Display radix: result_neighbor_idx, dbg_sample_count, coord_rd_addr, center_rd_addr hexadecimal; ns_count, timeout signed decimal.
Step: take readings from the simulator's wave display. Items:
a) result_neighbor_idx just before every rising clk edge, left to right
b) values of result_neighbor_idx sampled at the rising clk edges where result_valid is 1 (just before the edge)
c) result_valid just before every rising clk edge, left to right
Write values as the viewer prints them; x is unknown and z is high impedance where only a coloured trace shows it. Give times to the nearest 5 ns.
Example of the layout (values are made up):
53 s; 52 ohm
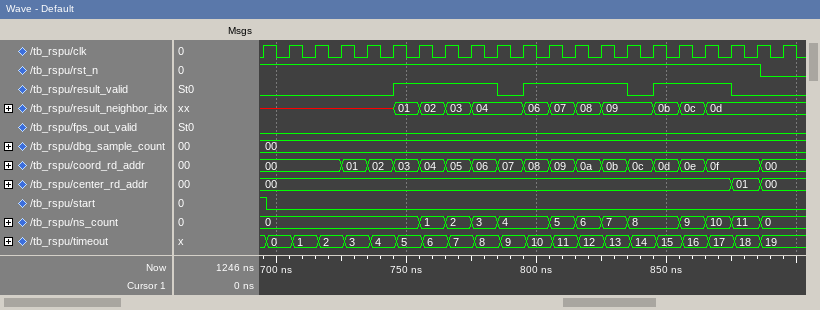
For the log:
x, x, x, x, x, x, 01, 02, 03, 04, 04, 06, 07, 08, 09, 09, 0b, 0c, 0d, 0d, 0d; 01, 02, 03, 04, 06, 07, 08, 09, 0b, 0c, 0d; 0 0 0 0 0 0 1 1 1 1 0 1 1 1 1 0 1 1 1 0 0
